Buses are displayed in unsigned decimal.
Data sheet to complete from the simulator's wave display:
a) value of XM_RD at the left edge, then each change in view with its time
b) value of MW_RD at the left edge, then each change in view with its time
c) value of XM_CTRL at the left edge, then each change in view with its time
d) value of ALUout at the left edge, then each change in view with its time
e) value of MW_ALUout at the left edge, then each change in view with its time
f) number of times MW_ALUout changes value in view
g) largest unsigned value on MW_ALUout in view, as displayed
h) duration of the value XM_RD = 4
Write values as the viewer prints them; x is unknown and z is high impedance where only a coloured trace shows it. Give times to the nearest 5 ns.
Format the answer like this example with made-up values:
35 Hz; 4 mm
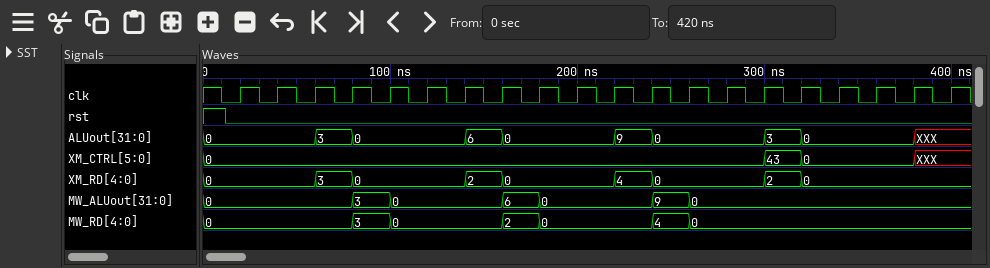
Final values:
0, 3 at 60 ns, 0 at 80 ns, 2 at 140 ns, 0 at 160 ns, 4 at 220 ns, 0 at 240 ns, 2 at 300 ns, 0 at 320 ns; 0, 3 at 80 ns, 0 at 100 ns, 2 at 160 ns, 0 at 180 ns, 4 at 240 ns, 0 at 260 ns; 0, 43 at 300 ns, 0 at 320 ns, XXX at 380 ns; 0, 3 at 60 ns, 0 at 80 ns, 6 at 140 ns, 0 at 160 ns, 9 at 220 ns, 0 at 240 ns, 3 at 300 ns, 0 at 320 ns, XXX at 380 ns; 0, 3 at 80 ns, 0 at 100 ns, 6 at 160 ns, 0 at 180 ns, 9 at 240 ns, 0 at 260 ns; 6; 9; 20 ns
